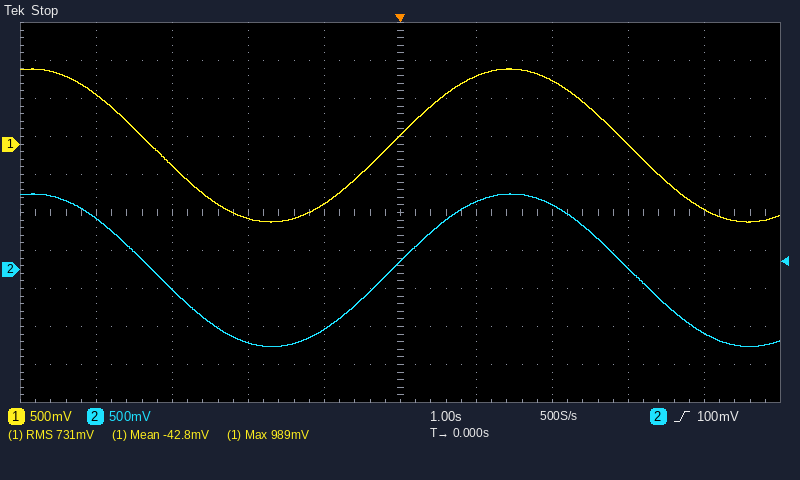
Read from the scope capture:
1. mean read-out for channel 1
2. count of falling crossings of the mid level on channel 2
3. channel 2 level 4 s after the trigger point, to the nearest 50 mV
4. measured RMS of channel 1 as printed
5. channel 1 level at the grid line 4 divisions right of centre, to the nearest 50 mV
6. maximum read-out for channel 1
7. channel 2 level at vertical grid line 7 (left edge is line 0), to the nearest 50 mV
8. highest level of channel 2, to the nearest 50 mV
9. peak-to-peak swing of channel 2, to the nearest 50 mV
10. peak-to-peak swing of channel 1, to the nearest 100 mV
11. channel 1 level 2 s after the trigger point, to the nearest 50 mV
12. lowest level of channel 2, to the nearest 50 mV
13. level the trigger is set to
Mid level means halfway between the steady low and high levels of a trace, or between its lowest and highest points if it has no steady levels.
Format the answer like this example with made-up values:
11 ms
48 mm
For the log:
-42.8 mV
2
-850 mV
731 mV
-850 mV
989 mV
850 mV
1.00 V
2.00 V
2.00 V
850 mV
-1.00 V
100 mV
